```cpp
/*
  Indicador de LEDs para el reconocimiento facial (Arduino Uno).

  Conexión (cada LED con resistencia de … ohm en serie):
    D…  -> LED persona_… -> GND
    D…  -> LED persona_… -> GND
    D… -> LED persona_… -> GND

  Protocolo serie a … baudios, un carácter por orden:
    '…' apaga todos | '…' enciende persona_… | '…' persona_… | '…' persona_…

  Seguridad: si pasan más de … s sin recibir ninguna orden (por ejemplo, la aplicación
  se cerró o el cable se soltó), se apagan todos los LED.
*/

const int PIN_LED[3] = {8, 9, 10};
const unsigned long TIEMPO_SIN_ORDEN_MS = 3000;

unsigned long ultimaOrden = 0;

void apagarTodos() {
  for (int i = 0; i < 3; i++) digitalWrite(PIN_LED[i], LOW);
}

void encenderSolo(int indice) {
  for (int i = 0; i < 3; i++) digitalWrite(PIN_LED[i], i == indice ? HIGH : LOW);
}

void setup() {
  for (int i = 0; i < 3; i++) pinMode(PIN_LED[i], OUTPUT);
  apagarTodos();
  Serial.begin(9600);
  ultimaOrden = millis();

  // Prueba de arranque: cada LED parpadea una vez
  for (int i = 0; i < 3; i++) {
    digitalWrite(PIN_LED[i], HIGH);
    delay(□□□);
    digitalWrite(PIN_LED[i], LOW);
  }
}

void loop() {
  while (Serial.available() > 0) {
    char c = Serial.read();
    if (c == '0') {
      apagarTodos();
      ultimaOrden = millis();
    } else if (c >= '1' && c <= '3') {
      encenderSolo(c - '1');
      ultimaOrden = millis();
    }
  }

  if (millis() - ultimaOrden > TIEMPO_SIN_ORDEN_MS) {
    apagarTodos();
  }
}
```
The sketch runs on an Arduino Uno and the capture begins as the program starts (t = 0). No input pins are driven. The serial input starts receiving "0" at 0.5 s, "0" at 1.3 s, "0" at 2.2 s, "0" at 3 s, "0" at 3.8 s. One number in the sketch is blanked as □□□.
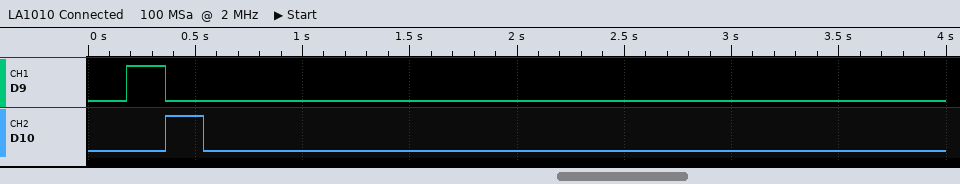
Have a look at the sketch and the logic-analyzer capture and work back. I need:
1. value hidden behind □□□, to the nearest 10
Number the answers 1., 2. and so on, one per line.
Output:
1. 180
